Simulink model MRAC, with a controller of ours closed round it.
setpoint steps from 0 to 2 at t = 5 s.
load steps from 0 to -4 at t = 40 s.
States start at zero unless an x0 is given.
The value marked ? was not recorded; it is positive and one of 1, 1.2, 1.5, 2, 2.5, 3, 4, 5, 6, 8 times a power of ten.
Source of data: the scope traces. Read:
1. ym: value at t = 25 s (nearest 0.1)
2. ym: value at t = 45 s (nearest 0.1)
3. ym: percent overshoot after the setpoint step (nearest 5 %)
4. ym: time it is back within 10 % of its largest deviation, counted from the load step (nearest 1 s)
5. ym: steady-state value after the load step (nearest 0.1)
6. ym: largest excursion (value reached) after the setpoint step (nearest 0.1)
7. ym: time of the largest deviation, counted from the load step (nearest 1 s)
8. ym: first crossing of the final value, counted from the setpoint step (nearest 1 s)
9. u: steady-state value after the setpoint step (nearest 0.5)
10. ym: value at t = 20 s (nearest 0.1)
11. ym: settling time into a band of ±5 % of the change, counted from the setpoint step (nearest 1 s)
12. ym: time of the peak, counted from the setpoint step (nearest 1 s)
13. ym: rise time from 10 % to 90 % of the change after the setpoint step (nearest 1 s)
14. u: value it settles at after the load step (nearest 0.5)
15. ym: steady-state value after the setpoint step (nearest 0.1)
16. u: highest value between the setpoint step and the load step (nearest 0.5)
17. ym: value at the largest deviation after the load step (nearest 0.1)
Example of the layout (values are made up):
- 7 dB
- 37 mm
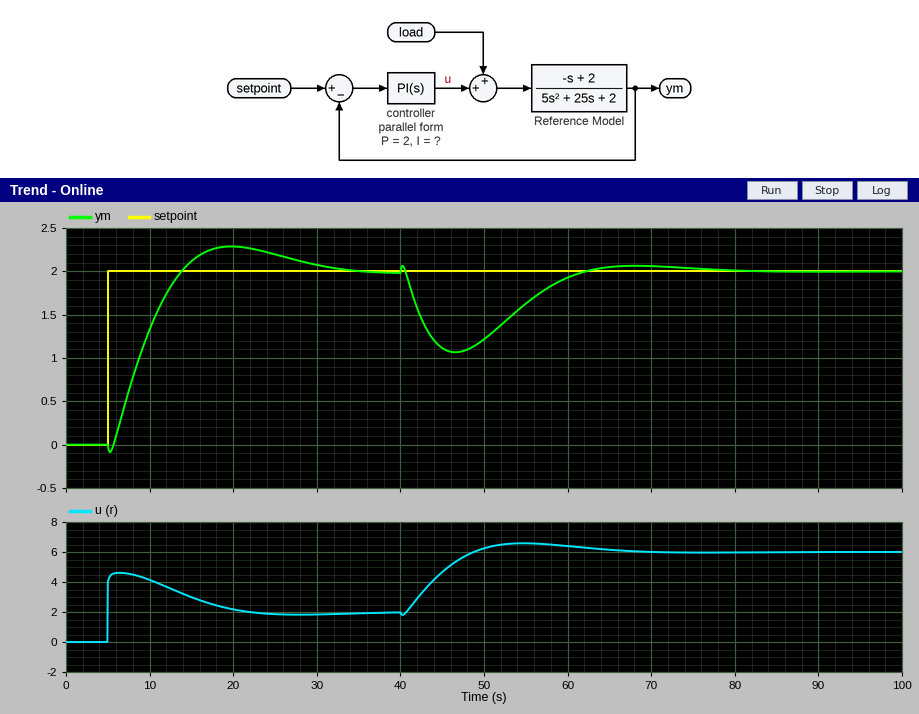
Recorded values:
- 2.2
- 1.1
- 15 %
- 20 s
- 2.0
- 2.3
- 7 s
- 9 s
- 2.0
- 2.3
- 24 s
- 15 s
- 6 s
- 6.0
- 2.0
- 4.5
- 1.1
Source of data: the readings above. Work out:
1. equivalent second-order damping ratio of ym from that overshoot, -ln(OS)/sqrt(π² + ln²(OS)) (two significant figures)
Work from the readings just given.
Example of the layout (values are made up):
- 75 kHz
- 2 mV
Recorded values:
- 0.52
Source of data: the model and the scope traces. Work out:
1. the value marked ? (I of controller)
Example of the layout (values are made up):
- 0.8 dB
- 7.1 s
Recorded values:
- 0.4
